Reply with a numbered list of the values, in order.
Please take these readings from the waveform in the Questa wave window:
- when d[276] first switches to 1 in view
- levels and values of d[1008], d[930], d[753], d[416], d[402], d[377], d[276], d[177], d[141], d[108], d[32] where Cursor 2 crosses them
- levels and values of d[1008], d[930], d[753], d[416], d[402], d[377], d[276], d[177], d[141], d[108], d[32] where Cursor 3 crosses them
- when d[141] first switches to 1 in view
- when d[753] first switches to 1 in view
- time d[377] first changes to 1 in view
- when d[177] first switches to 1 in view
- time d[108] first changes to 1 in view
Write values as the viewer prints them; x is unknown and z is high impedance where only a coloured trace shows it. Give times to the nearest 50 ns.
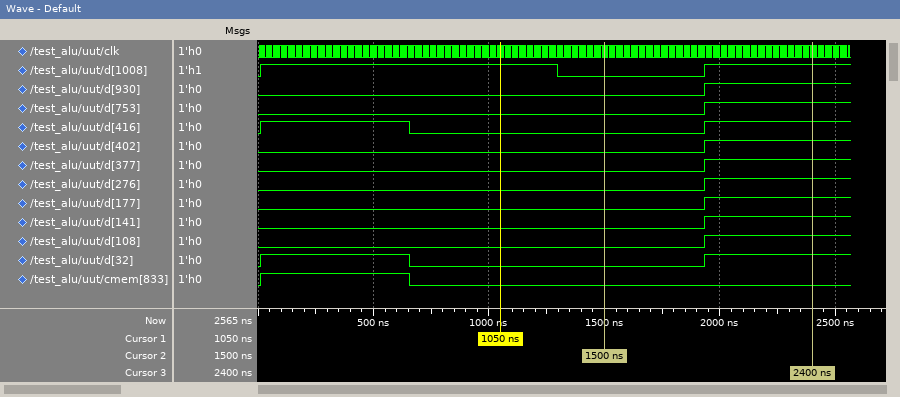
1. 1950 ns
2. d[1008]=0, d[930]=0, d[753]=0, d[416]=0, d[402]=0, d[377]=0, d[276]=0, d[177]=0, d[141]=0, d[108]=0, d[32]=0
3. d[1008]=1, d[930]=1, d[753]=1, d[416]=1, d[402]=1, d[377]=1, d[276]=1, d[177]=1, d[141]=1, d[108]=1, d[32]=1
4. 1950 ns
5. 1950 ns
6. 1950 ns
7. 1950 ns
8. 1950 ns
